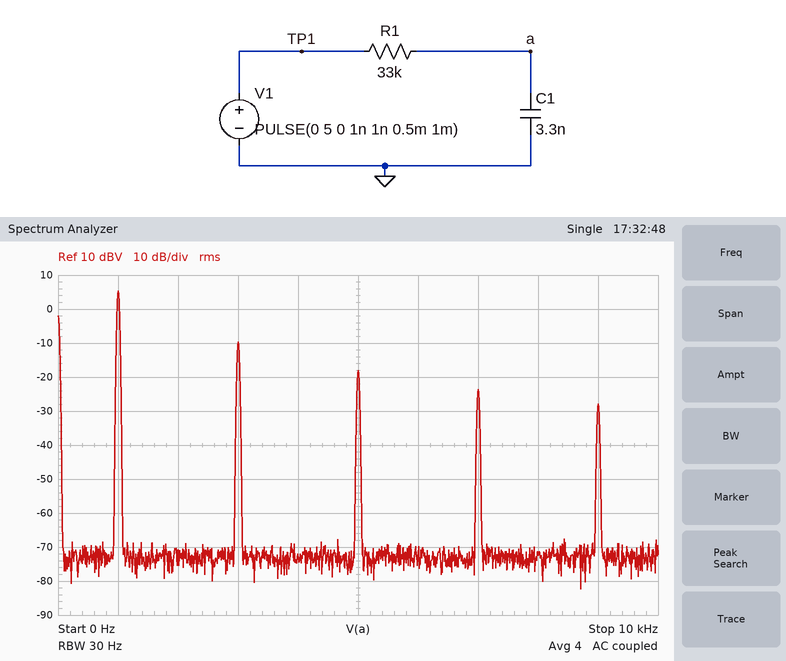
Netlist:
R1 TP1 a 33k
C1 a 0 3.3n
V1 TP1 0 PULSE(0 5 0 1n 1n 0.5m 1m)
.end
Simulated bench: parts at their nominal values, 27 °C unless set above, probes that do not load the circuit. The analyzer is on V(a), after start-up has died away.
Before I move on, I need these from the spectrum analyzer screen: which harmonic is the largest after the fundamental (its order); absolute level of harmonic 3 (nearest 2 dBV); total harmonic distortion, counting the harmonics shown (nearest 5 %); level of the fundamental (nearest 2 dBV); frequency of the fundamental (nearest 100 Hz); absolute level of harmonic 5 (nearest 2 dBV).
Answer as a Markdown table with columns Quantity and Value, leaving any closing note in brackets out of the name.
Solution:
| Quantity | Value |
|---|---|
| which harmonic is the largest after the fundamental | 3 |
| absolute level of harmonic 3 | -10 dBV |
| total harmonic distortion, counting the harmonics shown | 20 % |
| level of the fundamental | 6 dBV |
| frequency of the fundamental | 1.0 kHz |
| absolute level of harmonic 5 | -18 dBV |
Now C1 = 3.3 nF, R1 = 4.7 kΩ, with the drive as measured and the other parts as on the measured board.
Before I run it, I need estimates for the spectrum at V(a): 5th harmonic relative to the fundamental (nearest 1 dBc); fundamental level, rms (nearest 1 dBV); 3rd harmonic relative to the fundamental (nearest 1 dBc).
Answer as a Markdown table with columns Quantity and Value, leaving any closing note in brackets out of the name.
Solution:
| Quantity | Value |
|---|---|
| 5th harmonic relative to the fundamental | -15 dBc |
| fundamental level, rms | 7 dBV |
| 3rd harmonic relative to the fundamental | -10 dBc |
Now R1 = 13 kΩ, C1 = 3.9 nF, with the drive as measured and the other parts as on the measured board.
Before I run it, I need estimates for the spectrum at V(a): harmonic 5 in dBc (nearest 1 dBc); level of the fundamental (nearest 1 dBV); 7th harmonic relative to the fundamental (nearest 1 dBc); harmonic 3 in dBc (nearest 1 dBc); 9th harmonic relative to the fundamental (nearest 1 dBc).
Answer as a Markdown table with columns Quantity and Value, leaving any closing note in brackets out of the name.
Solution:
| Quantity | Value |
|---|---|
| harmonic 5 in dBc | -19 dBc |
| level of the fundamental | 7 dBV |
| 7th harmonic relative to the fundamental | -24 dBc |
| harmonic 3 in dBc | -12 dBc |
| 9th harmonic relative to the fundamental | -28 dBc |
